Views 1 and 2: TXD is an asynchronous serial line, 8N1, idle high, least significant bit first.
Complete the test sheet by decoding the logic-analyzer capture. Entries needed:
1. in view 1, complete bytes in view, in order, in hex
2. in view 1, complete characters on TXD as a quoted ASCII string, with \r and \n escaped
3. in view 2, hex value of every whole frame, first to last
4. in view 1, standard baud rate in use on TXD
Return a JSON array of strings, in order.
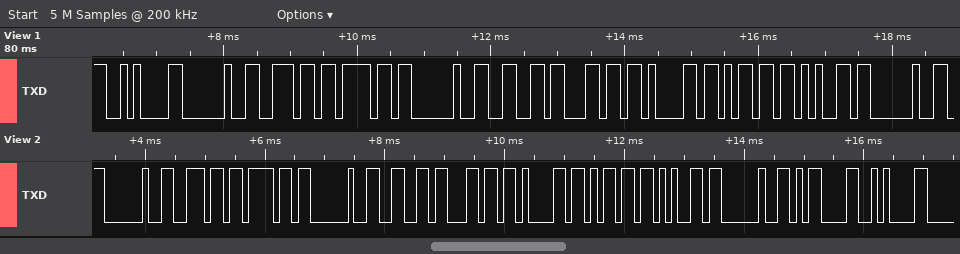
["0x0A 0x20 0x6E 0x6F 0x20 0x66 0x6C 0x61 0x6D 0x65 0x20", "\"\\n no flame \"", "20 6E 6F 20 66 6C 61 6D 65 20 0D 0A", "9600 baud"]
